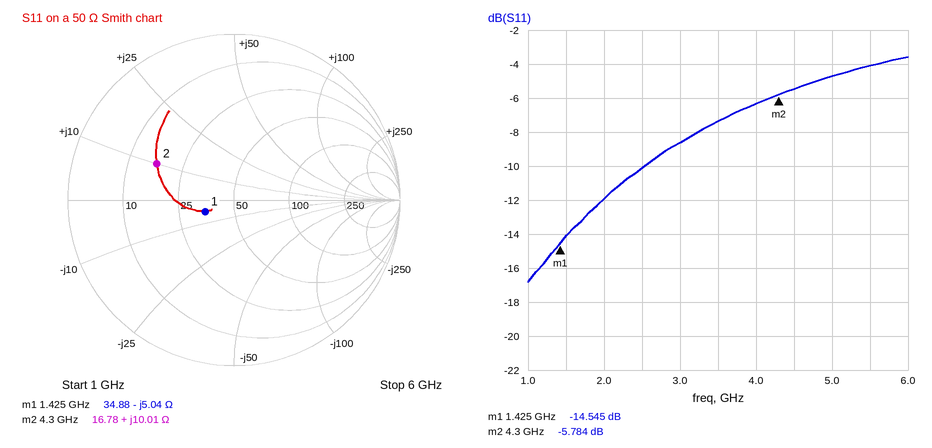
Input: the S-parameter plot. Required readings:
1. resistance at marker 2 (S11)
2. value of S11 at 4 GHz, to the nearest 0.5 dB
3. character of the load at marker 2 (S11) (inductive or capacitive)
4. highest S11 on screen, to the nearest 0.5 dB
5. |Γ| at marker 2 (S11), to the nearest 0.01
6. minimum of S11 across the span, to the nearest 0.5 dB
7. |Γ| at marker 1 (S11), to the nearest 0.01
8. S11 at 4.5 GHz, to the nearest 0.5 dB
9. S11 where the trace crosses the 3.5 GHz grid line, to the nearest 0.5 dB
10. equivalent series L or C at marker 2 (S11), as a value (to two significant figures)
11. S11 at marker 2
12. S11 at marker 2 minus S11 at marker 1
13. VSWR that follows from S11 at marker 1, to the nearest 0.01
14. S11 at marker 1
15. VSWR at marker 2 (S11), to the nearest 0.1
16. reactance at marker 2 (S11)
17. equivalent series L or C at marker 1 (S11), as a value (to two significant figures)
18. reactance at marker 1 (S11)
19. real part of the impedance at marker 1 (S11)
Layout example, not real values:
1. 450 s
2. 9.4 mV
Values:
1. 16.78 Ω
2. -6.5 dB
3. inductive
4. -3.5 dB
5. 0.51
6. -17.0 dB
7. 0.19
8. -5.5 dB
9. -7.5 dB
10. 370 pH
11. -5.784 dB
12. 8.761 dB
13. 1.46
14. -14.545 dB
15. 3.1
16. +10.01 Ω
17. 22 pF
18. -5.04 Ω
19. 34.88 Ω
